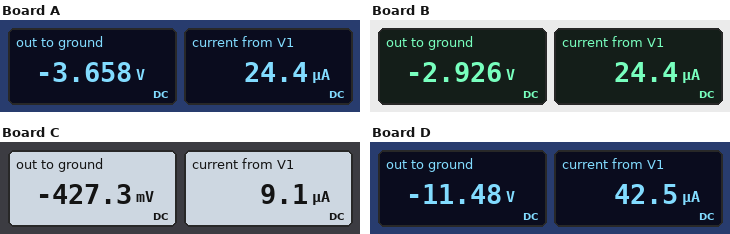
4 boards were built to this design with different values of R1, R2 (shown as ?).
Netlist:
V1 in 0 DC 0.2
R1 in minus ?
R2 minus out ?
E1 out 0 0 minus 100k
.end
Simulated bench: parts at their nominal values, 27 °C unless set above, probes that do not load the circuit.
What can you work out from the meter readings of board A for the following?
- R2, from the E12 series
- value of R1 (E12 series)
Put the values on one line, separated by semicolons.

150 kΩ; 8.2 kΩ
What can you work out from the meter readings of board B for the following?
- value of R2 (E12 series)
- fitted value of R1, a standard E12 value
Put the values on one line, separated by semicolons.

120 kΩ; 8.2 kΩ
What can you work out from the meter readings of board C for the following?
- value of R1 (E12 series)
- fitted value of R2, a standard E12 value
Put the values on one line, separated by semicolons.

22 kΩ; 47 kΩ
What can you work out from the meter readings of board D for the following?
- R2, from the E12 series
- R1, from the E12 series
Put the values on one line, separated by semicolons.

270 kΩ; 4.7 kΩ
